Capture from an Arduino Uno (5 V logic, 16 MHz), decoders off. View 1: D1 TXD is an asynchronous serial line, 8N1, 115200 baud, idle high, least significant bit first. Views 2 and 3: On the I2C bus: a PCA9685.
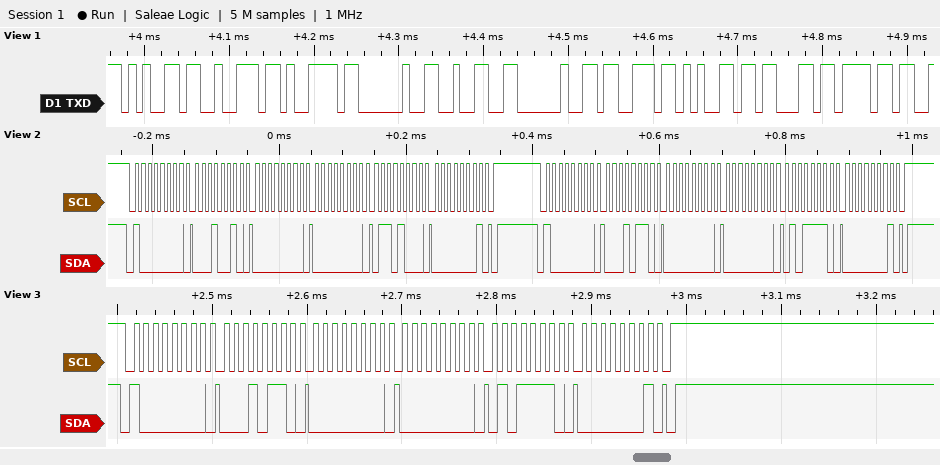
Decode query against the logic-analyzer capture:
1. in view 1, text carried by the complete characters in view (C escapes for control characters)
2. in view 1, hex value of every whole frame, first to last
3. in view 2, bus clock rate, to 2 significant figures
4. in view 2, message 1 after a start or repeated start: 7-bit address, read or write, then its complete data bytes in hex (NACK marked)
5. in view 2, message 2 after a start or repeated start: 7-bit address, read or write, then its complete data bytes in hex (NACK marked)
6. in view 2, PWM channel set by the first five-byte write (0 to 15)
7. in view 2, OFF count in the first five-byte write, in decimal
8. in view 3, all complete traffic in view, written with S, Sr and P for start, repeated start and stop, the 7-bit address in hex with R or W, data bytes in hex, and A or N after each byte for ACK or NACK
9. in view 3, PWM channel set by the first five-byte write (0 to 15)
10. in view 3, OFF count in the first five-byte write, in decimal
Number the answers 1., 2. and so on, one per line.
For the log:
1. "ery 2 seco"
2. 0x65 0x72 0x79 0x20 0x32 0x20 0x73 0x65 0x63 0x6F
3. 100 kHz
4. 0x40 write: 12 00 00 68 01
5. 0x40 write: 16 00 00 5E 01
6. 3
7. 360
8. S 40W A 16 A 00 A 00 A 5E A 01 A P
9. 4
10. 350
